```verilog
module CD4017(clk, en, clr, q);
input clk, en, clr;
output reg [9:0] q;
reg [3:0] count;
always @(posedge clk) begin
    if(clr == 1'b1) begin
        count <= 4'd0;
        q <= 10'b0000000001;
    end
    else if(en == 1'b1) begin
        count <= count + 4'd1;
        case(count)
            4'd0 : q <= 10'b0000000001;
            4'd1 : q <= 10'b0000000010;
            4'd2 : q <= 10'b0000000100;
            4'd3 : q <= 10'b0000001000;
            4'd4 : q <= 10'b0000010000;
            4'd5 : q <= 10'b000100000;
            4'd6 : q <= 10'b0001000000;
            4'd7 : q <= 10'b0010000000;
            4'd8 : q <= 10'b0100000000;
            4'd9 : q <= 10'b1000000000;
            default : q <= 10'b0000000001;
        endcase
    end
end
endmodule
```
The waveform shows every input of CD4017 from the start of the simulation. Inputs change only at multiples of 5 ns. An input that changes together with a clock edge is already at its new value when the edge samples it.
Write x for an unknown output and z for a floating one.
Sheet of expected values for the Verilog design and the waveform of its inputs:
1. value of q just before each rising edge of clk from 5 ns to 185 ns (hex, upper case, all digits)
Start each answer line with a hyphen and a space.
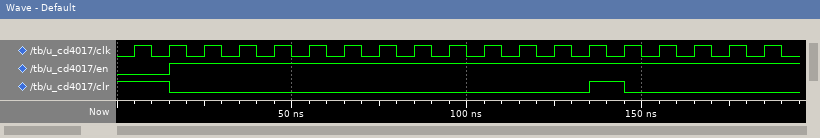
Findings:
- x, 001, 001, 002, 004, 008, 010, 020, 040, 080, 100, 200, 001, 001, 001, 001, 002, 004, 008
